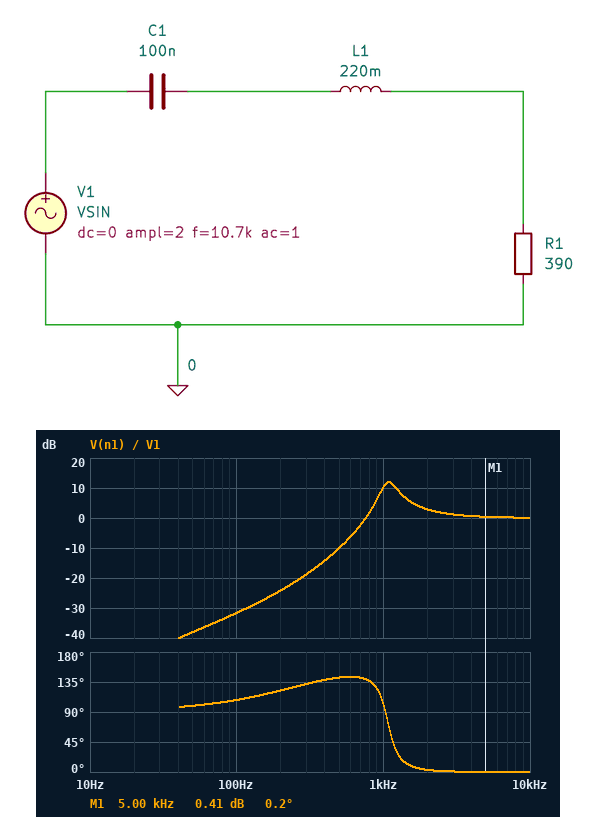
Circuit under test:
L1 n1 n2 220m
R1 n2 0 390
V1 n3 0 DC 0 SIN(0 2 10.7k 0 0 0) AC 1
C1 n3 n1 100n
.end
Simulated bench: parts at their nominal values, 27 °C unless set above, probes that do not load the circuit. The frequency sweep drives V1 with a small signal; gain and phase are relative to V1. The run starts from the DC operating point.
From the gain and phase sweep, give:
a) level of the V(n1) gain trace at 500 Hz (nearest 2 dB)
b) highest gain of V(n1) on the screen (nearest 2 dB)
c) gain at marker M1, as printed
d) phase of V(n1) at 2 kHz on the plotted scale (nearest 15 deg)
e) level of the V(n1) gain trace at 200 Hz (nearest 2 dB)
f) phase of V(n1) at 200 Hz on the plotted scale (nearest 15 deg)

-10 dB
12 dB
0.41 dB
0 deg
-24 dB
120 deg
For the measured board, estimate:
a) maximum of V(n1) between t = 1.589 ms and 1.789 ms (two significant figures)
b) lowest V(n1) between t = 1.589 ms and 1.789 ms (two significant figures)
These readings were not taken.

2.1 V
-2.0 V
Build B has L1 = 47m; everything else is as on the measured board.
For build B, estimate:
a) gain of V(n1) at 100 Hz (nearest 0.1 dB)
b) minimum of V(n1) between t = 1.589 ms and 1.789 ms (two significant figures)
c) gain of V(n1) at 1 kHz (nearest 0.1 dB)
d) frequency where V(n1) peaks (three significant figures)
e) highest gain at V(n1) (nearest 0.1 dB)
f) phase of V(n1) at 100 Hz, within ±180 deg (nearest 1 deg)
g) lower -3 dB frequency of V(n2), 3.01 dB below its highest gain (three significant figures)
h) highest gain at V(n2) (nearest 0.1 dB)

-32.2 dB
-2.1 V
-8.8 dB
2.48 kHz
6.3 dB
93 deg
1.75 kHz
0 dB
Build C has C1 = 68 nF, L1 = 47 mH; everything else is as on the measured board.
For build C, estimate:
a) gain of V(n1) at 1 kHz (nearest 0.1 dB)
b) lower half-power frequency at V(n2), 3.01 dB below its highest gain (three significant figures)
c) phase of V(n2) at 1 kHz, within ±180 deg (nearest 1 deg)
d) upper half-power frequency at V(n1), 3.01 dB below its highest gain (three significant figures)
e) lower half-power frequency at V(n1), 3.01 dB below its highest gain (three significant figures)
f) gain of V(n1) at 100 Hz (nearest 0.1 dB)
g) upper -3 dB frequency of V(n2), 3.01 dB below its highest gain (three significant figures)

-12.6 dB
2.23 kHz
79 deg
4.10 kHz
2.39 kHz
-35.5 dB
3.55 kHz
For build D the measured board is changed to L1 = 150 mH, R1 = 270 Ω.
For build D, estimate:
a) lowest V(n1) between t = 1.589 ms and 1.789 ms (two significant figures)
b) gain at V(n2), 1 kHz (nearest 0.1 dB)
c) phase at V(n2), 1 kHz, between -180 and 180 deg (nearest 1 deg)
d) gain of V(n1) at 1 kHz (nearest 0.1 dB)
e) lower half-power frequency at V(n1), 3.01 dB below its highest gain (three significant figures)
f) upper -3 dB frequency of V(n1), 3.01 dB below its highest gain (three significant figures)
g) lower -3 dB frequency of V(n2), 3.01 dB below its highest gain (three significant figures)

-2.1 V
-8.3 dB
67 deg
2.9 dB
1.19 kHz
1.49 kHz
1.16 kHz
